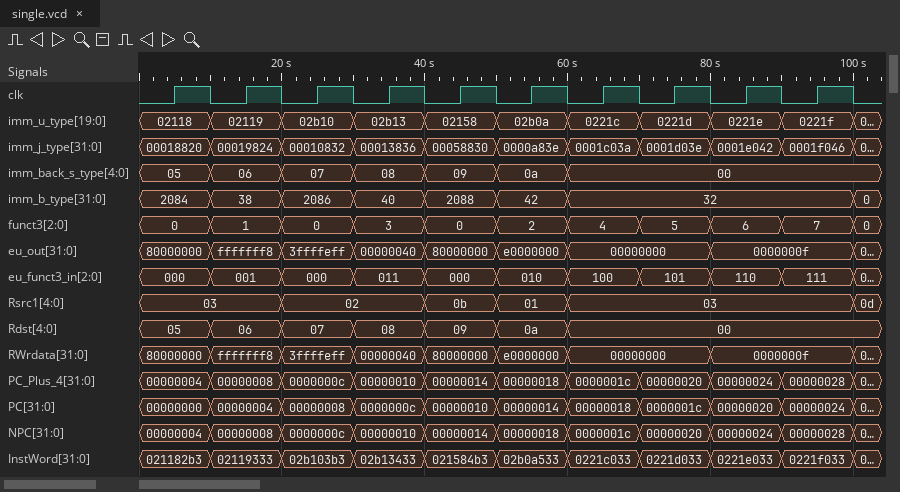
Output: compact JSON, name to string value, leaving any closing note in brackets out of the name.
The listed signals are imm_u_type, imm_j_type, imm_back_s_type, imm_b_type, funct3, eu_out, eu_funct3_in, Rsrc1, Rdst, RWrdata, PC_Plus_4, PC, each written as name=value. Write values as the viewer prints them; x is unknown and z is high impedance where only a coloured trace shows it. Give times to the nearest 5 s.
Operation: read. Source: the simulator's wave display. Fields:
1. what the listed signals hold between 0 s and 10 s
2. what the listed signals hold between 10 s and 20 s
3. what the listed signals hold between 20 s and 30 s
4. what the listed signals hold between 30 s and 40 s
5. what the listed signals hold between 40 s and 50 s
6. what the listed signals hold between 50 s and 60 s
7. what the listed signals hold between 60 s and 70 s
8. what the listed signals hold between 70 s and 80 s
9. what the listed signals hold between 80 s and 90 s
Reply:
{"what the listed signals hold between 0 s and 10 s": "imm_u_type=02118, imm_j_type=00018820, imm_back_s_type=05, imm_b_type=2084, funct3=0, eu_out=80000000, eu_funct3_in=000, Rsrc1=03, Rdst=05, RWrdata=80000000, PC_Plus_4=00000004, PC=00000000", "what the listed signals hold between 10 s and 20 s": "imm_u_type=02119, imm_j_type=00019824, imm_back_s_type=06, imm_b_type=38, funct3=1, eu_out=fffffff8, eu_funct3_in=001, Rsrc1=03, Rdst=06, RWrdata=fffffff8, PC_Plus_4=00000008, PC=00000004", "what the listed signals hold between 20 s and 30 s": "imm_u_type=02b10, imm_j_type=00010832, imm_back_s_type=07, imm_b_type=2086, funct3=0, eu_out=3ffffeff, eu_funct3_in=000, Rsrc1=02, Rdst=07, RWrdata=3ffffeff, PC_Plus_4=0000000c, PC=00000008", "what the listed signals hold between 30 s and 40 s": "imm_u_type=02b13, imm_j_type=00013836, imm_back_s_type=08, imm_b_type=40, funct3=3, eu_out=00000040, eu_funct3_in=011, Rsrc1=02, Rdst=08, RWrdata=00000040, PC_Plus_4=00000010, PC=0000000c", "what the listed signals hold between 40 s and 50 s": "imm_u_type=02158, imm_j_type=00058830, imm_back_s_type=09, imm_b_type=2088, funct3=0, eu_out=80000000, eu_funct3_in=000, Rsrc1=0b, Rdst=09, RWrdata=80000000, PC_Plus_4=00000014, PC=00000010", "what the listed signals hold between 50 s and 60 s": "imm_u_type=02b0a, imm_j_type=0000a83e, imm_back_s_type=0a, imm_b_type=42, funct3=2, eu_out=e0000000, eu_funct3_in=010, Rsrc1=01, Rdst=0a, RWrdata=e0000000, PC_Plus_4=00000018, PC=00000014", "what the listed signals hold between 60 s and 70 s": "imm_u_type=0221c, imm_j_type=0001c03a, imm_back_s_type=00, imm_b_type=32, funct3=4, eu_out=00000000, eu_funct3_in=100, Rsrc1=03, Rdst=00, RWrdata=00000000, PC_Plus_4=0000001c, PC=00000018", "what the listed signals hold between 70 s and 80 s": "imm_u_type=0221d, imm_j_type=0001d03e, imm_back_s_type=00, imm_b_type=32, funct3=5, eu_out=00000000, eu_funct3_in=101, Rsrc1=03, Rdst=00, RWrdata=00000000, PC_Plus_4=00000020, PC=0000001c", "what the listed signals hold between 80 s and 90 s": "imm_u_type=0221e, imm_j_type=0001e042, imm_back_s_type=00, imm_b_type=32, funct3=6, eu_out=0000000f, eu_funct3_in=110, Rsrc1=03, Rdst=00, RWrdata=0000000f, PC_Plus_4=00000024, PC=00000020"}
